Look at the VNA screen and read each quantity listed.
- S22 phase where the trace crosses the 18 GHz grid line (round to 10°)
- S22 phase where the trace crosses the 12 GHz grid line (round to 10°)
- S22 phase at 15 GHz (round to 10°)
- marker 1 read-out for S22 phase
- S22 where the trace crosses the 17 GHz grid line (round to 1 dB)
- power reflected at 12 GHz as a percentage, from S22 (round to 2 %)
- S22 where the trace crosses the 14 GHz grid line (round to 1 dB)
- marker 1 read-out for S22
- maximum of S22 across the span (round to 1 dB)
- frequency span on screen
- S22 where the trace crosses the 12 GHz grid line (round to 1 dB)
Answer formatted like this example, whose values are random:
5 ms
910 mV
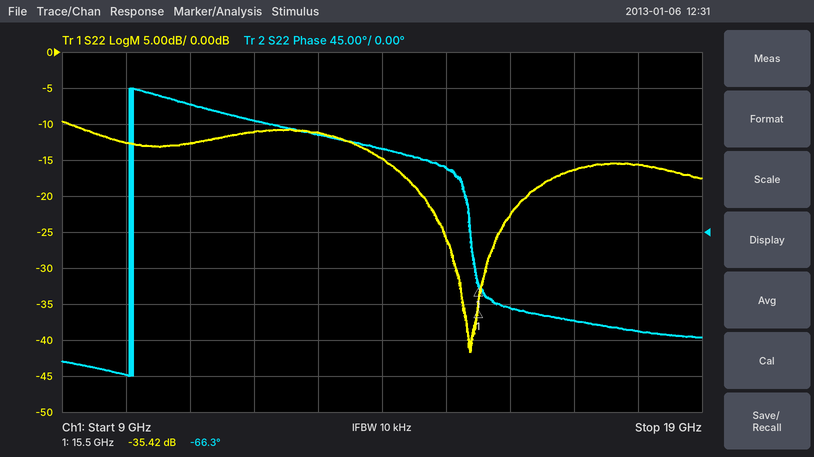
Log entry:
-120°
140°
80°
-66.3°
-16 dB
8 %
-15 dB
-35.42 dB
-10 dB
10 GHz
-11 dB
